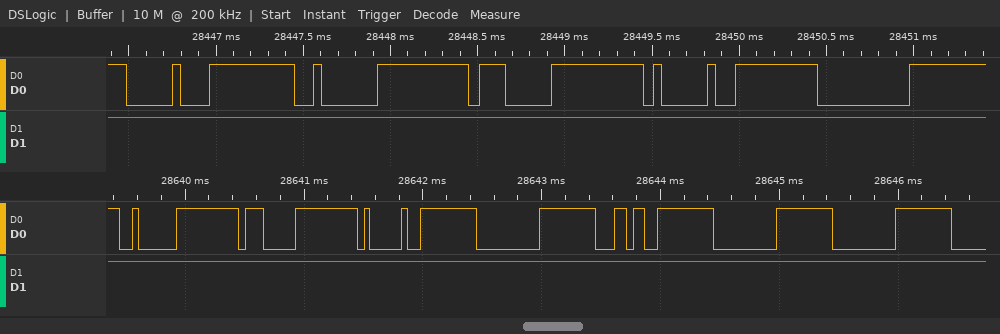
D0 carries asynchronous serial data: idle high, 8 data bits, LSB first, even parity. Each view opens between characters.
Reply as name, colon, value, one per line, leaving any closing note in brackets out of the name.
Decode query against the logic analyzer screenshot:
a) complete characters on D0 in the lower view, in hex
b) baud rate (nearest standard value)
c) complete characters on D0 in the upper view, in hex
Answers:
complete characters on D0 in the lower view, in hex: 02, 07, 41, 00, 6C, 00, 00
baud rate: 19200 baud
complete characters on D0 in the upper view, in hex: 10, 02, 07, 41, 00
